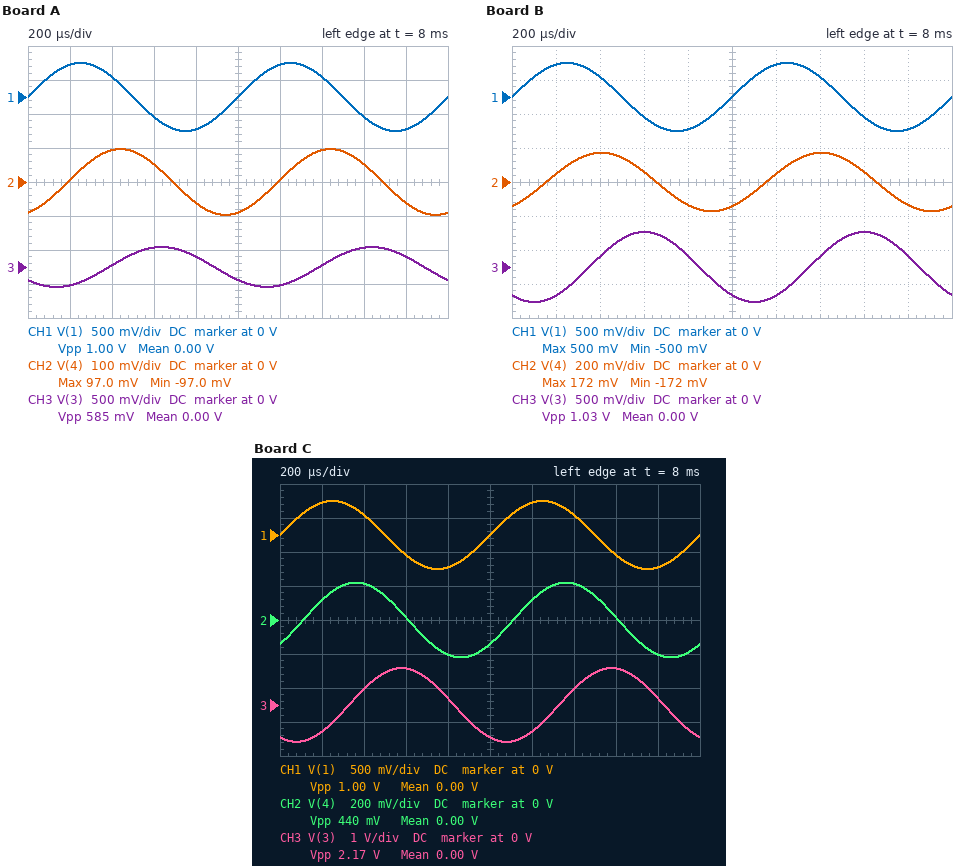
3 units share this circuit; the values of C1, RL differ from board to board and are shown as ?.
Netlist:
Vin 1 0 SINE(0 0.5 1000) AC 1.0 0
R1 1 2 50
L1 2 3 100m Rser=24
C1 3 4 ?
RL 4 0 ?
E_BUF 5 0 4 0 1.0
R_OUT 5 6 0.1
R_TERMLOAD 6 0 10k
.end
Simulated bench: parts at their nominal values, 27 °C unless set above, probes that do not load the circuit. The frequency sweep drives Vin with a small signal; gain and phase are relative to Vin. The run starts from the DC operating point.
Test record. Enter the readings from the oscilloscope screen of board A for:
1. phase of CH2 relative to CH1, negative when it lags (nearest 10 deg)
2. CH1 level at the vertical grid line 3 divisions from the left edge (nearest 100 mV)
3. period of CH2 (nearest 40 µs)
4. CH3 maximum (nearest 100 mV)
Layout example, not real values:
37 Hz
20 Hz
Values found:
-70 deg
-300 mV
1.00 ms
300 mV
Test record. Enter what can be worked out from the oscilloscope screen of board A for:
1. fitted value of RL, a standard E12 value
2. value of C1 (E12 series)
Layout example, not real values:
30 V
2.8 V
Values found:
82 Ω
680 nF
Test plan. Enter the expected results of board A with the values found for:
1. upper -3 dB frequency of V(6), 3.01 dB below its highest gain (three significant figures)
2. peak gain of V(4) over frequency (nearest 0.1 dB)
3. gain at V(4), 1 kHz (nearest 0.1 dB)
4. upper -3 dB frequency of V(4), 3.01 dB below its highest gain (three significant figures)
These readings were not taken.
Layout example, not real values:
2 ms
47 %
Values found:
747 Hz
-5.6 dB
-14.3 dB
747 Hz
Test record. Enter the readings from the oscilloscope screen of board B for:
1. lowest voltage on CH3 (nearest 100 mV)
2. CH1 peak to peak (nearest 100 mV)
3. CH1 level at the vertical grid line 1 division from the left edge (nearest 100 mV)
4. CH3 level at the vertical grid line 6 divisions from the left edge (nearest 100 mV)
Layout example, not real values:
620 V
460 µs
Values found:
-500 mV
1.0 V
500 mV
-400 mV
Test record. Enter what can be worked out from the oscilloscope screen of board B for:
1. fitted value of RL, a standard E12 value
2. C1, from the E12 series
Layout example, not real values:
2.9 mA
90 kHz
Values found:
120 Ω
470 nF
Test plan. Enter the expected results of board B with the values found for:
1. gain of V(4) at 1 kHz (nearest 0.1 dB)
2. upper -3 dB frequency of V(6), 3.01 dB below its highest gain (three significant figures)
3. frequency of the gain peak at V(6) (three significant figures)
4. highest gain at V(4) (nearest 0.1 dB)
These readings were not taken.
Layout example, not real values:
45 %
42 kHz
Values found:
-9.3 dB
905 Hz
734 Hz
-4.2 dB
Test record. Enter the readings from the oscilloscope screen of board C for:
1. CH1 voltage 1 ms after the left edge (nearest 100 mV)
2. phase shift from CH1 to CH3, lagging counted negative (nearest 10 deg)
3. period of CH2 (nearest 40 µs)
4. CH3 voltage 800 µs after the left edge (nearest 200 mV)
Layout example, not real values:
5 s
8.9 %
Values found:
0 V
-120 deg
1.00 ms
200 mV
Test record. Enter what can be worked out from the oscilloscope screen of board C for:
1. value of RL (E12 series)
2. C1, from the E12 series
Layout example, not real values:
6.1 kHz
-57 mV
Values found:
100 Ω
330 nF
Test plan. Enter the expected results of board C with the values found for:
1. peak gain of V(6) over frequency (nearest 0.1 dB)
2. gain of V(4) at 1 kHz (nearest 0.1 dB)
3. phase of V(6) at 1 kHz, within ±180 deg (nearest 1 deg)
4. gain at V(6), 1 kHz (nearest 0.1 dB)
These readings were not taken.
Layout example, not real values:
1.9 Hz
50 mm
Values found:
-4.8 dB
-7.1 dB
-40 deg
-7.1 dB
